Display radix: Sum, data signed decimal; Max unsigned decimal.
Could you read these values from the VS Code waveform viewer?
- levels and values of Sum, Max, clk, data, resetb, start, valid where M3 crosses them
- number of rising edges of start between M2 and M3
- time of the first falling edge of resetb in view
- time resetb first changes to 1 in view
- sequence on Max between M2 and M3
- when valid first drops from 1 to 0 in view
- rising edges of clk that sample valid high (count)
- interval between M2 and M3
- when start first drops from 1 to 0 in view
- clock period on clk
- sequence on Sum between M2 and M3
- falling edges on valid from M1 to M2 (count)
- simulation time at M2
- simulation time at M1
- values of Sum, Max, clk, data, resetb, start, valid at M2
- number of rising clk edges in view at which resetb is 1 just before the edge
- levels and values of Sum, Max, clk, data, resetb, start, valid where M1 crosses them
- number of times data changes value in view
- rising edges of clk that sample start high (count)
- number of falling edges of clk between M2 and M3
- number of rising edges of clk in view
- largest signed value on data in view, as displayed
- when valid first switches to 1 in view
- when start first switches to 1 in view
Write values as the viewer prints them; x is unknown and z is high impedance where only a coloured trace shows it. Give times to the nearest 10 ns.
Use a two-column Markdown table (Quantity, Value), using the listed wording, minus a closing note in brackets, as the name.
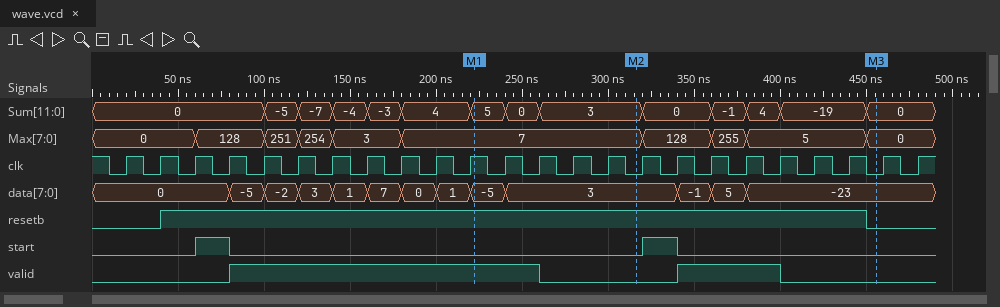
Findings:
| Quantity | Value |
|---|---|
| levels and values of Sum, Max, clk, data, resetb, start, valid where M3 crosses them | Sum=0, Max=0, clk=0, data=-23, resetb=0, start=0, valid=0 |
| number of rising edges of start between M2 and M3 | 1 |
| time of the first falling edge of resetb in view | 450 ns |
| time resetb first changes to 1 in view | 40 ns |
| sequence on Max between M2 and M3 | 7, 128, 255, 5, 0 |
| when valid first drops from 1 to 0 in view | 260 ns |
| rising edges of clk that sample valid high | 12 |
| interval between M2 and M3 | 140 ns |
| when start first drops from 1 to 0 in view | 80 ns |
| clock period on clk | 20 ns |
| sequence on Sum between M2 and M3 | 3, 0, -1, 4, -19, 0 |
| falling edges on valid from M1 to M2 | 1 |
| simulation time at M2 | 320 ns |
| simulation time at M1 | 220 ns |
| values of Sum, Max, clk, data, resetb, start, valid at M2 | Sum=3, Max=7, clk=0, data=3, resetb=1, start=0, valid=0 |
| number of rising clk edges in view at which resetb is 1 just before the edge | 20 |
| levels and values of Sum, Max, clk, data, resetb, start, valid where M1 crosses them | Sum=5, Max=7, clk=1, data=-5, resetb=1, start=0, valid=1 |
| number of times data changes value in view | 12 |
| rising edges of clk that sample start high | 2 |
| number of falling edges of clk between M2 and M3 | 7 |
| number of rising edges of clk in view | 24 |
| largest signed value on data in view, as displayed | 7 |
| when valid first switches to 1 in view | 80 ns |
| when start first switches to 1 in view | 60 ns |
